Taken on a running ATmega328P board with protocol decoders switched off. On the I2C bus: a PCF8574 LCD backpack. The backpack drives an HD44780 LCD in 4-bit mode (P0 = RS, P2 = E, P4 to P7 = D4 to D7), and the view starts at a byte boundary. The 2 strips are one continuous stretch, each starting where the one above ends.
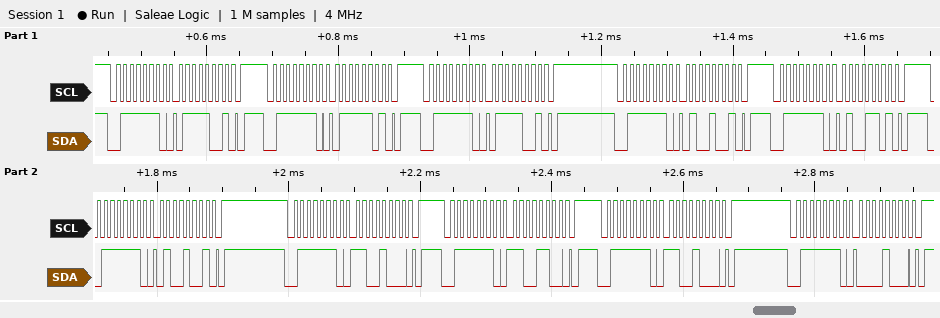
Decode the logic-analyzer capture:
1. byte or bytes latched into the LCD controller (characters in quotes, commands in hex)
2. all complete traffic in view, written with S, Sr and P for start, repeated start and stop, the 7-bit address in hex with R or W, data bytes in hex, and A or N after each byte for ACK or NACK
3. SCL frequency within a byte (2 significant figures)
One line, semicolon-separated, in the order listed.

't'; S 3FW A 79 A P S 3FW A 7D A P S 3FW A 79 A P S 3FW A 49 A P S 3FW A 4D A P S 3FW A 49 A P S 3FW A C8 A P S 3FW A CC A P S 3FW A C8 A P S 3FW A 08 A P; 100 kHz
